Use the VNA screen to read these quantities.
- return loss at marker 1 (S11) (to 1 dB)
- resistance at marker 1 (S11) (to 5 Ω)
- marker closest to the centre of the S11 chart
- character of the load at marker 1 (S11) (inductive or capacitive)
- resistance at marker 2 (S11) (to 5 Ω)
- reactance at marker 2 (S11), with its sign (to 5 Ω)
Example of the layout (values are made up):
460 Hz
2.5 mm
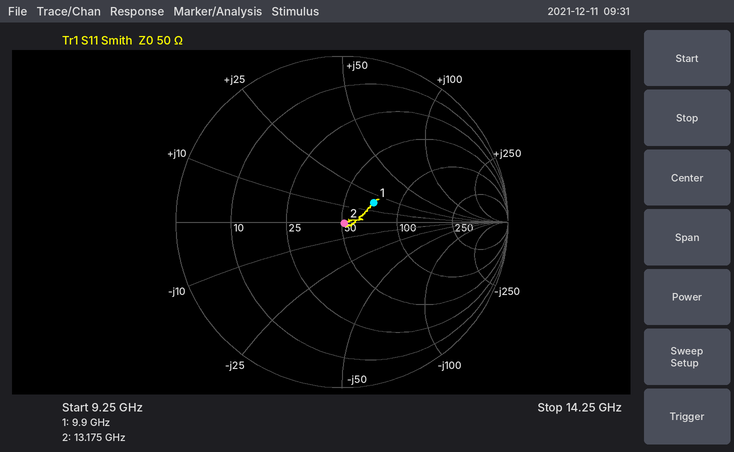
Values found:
13 dB
70 Ω
marker 2
inductive
50 Ω
0 Ω
